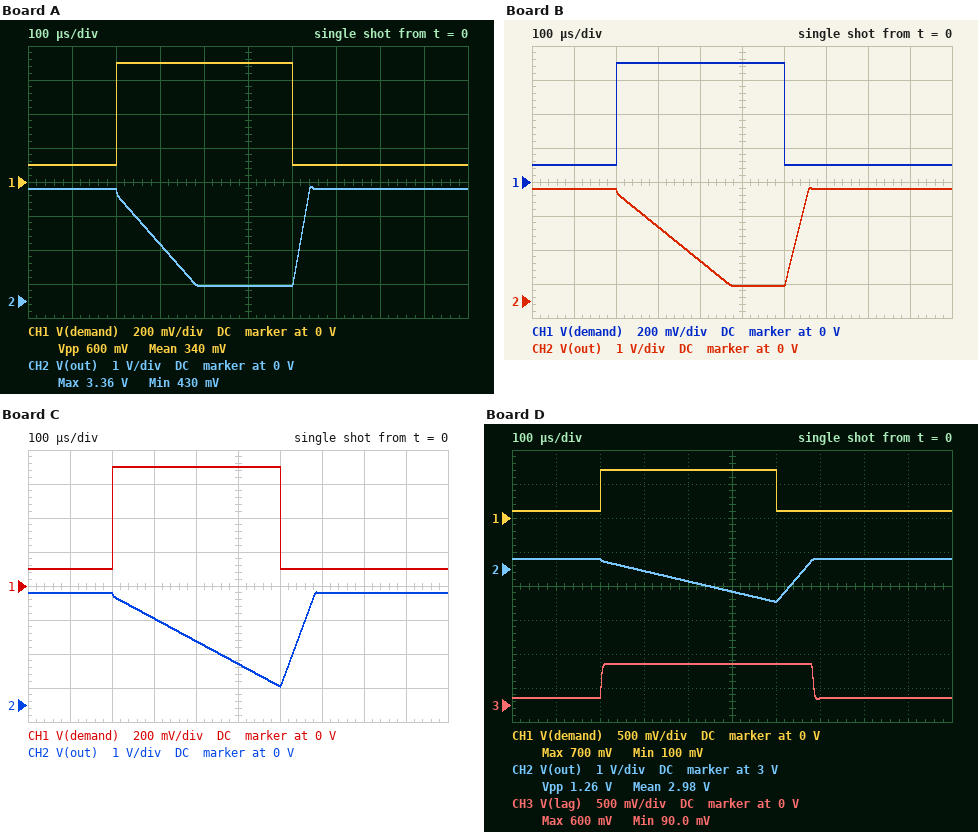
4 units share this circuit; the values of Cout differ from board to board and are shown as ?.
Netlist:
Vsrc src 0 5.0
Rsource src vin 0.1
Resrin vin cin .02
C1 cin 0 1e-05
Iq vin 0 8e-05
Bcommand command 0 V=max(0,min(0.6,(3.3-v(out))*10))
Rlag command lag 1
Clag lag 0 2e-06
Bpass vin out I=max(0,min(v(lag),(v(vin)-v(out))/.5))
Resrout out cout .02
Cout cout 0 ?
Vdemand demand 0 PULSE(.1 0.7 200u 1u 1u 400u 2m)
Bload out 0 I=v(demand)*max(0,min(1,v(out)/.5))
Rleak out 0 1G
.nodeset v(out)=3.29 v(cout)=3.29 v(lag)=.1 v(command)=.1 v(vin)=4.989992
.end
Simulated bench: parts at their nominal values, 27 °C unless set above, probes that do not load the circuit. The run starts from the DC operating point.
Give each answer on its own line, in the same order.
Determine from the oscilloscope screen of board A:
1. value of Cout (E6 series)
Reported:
6.8 µF
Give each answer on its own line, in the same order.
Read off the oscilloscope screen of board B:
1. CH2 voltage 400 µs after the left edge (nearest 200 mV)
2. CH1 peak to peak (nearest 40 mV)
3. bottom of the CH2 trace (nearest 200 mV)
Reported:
1.2 V
600 mV
400 mV
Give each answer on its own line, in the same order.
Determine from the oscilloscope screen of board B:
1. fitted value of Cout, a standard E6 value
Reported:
10 µF
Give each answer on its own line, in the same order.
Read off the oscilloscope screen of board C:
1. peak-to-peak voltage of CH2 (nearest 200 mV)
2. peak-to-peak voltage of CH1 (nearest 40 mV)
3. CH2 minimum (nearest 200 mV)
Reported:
2.8 V
600 mV
600 mV
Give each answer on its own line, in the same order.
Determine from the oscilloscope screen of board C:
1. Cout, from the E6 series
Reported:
15 µF
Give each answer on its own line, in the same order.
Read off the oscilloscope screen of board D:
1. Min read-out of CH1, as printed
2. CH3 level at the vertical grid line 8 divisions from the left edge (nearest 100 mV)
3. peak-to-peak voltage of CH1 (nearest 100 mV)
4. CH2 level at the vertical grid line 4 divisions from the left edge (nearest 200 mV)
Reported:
100 mV
100 mV
600 mV
2.6 V
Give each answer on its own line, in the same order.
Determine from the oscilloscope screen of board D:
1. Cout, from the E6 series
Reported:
33 µF
